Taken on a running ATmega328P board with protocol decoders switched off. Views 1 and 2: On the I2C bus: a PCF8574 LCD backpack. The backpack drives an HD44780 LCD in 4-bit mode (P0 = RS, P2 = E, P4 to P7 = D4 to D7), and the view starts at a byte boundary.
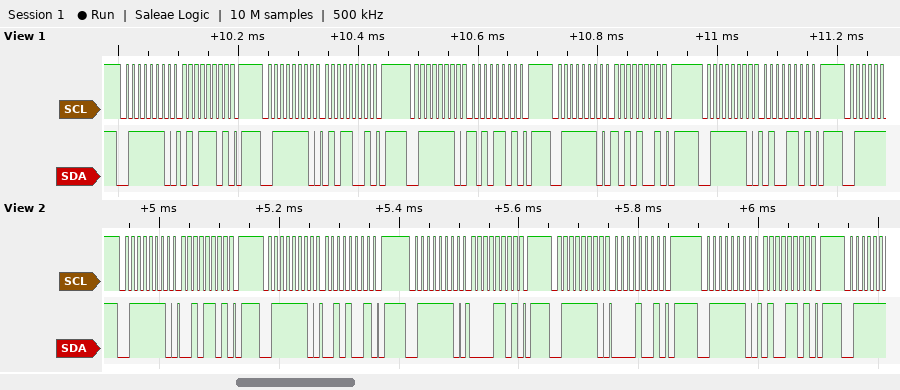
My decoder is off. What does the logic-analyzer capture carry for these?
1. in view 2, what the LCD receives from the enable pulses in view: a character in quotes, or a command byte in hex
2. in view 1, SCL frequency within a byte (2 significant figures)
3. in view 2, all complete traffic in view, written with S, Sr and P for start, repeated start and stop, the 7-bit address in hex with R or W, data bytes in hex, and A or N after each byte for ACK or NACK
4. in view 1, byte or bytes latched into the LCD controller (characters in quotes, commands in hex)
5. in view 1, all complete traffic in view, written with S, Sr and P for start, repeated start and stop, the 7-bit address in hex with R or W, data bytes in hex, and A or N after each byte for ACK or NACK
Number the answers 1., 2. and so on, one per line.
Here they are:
1. ' '
2. 100 kHz
3. S 3FW A 2D A P S 3FW A 29 A P S 3FW A 0D A P S 3FW A 09 A P S 3FW A 4D A P
4. 'Z'
5. S 3FW A 5D A P S 3FW A 59 A P S 3FW A AD A P S 3FW A A9 A P S 3FW A 4D A P
